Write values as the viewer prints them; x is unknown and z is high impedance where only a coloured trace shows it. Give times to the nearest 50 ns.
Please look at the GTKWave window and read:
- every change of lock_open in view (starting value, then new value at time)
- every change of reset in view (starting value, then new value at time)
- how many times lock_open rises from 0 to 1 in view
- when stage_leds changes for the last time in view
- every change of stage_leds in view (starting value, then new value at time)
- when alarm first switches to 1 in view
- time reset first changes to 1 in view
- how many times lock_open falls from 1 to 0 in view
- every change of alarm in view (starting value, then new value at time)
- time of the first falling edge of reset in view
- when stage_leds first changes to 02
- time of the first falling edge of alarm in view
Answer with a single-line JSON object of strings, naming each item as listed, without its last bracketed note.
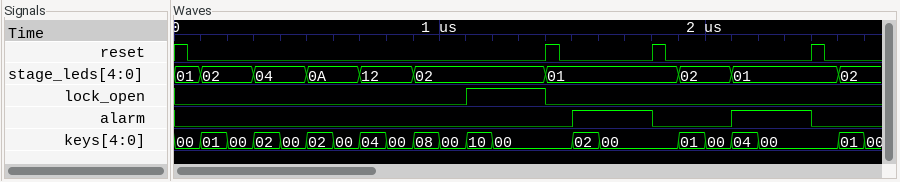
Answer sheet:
{"every change of lock_open in view": "0, 1 at 1100 ns, 0 at 1400 ns", "every change of reset in view": "1, 0 at 50 ns, 1 at 1400 ns, 0 at 1450 ns, 1 at 1800 ns, 0 at 1850 ns, 1 at 2400 ns, 0 at 2450 ns", "how many times lock_open rises from 0 to 1 in view": "1", "when stage_leds changes for the last time in view": "2500 ns", "every change of stage_leds in view": "01, 02 at 100 ns, 04 at 300 ns, 0A at 500 ns, 12 at 700 ns, 02 at 900 ns, 01 at 1400 ns, 02 at 1900 ns, 01 at 2100 ns, 02 at 2500 ns", "when alarm first switches to 1 in view": "1500 ns", "time reset first changes to 1 in view": "1400 ns", "how many times lock_open falls from 1 to 0 in view": "1", "every change of alarm in view": "0, 1 at 1500 ns, 0 at 1800 ns, 1 at 2100 ns, 0 at 2400 ns", "time of the first falling edge of reset in view": "50 ns", "when stage_leds first changes to 02": "100 ns", "time of the first falling edge of alarm in view": "1800 ns"}
